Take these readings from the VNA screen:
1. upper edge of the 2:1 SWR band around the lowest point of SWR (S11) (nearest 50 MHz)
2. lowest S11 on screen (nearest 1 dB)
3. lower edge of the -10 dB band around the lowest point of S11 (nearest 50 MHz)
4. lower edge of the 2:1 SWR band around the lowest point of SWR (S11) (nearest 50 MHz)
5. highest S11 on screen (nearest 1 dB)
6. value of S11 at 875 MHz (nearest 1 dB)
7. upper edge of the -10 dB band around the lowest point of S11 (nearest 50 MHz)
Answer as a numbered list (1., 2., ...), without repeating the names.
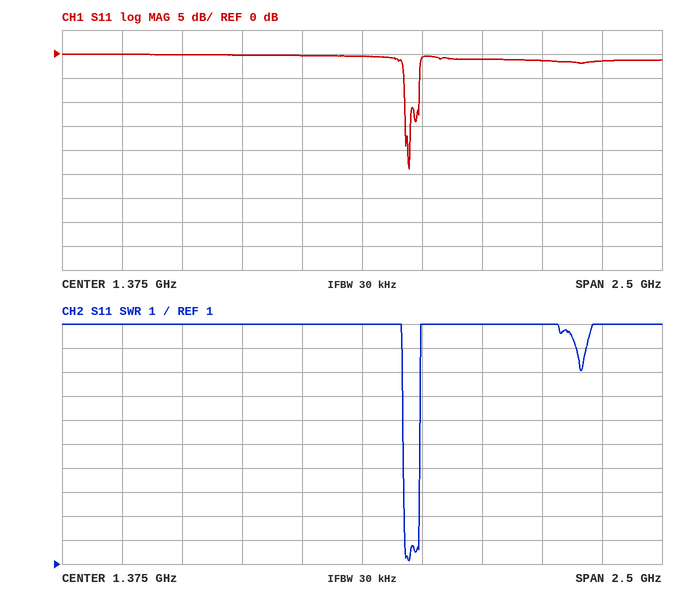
1. 1.60 GHz
2. -24 dB
3. 1.55 GHz
4. 1.55 GHz
5. 0 dB
6. 0 dB
7. 1.60 GHz
